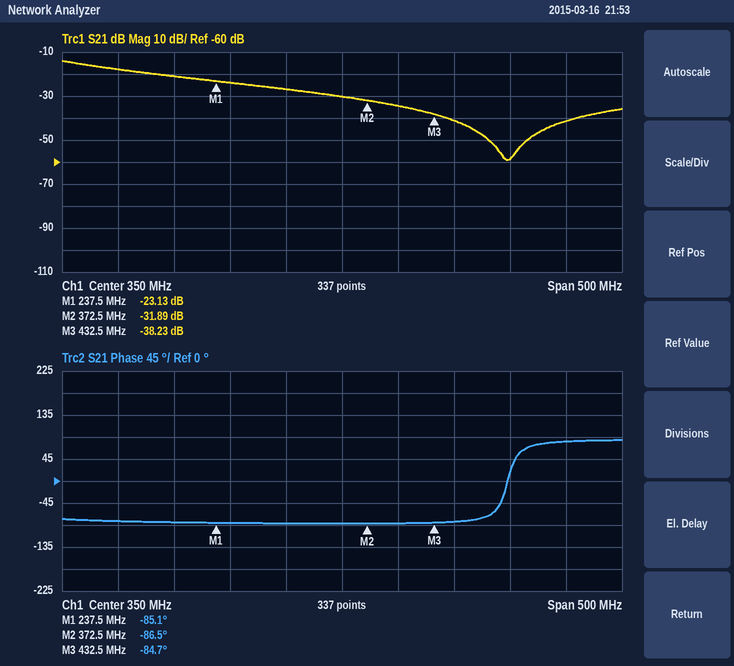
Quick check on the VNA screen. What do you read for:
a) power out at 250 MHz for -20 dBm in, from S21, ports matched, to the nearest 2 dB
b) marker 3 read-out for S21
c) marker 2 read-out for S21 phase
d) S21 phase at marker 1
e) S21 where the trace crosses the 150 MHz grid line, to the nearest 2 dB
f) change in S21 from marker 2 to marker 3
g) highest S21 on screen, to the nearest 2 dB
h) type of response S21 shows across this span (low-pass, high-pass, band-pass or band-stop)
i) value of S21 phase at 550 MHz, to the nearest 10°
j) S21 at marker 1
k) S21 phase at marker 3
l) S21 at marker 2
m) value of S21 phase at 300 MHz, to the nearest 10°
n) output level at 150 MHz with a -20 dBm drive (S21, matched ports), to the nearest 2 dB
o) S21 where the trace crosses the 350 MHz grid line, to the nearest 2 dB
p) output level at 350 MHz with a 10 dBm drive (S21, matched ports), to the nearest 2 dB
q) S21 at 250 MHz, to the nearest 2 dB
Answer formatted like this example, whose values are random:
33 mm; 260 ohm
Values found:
-44 dBm; -38.23 dB; -86.5°; -85.1°; -18 dB; -6.34 dB; -14 dB; low-pass; 80°; -23.13 dB; -84.7°; -31.89 dB; -90°; -38 dBm; -30 dB; -20 dBm; -24 dB
